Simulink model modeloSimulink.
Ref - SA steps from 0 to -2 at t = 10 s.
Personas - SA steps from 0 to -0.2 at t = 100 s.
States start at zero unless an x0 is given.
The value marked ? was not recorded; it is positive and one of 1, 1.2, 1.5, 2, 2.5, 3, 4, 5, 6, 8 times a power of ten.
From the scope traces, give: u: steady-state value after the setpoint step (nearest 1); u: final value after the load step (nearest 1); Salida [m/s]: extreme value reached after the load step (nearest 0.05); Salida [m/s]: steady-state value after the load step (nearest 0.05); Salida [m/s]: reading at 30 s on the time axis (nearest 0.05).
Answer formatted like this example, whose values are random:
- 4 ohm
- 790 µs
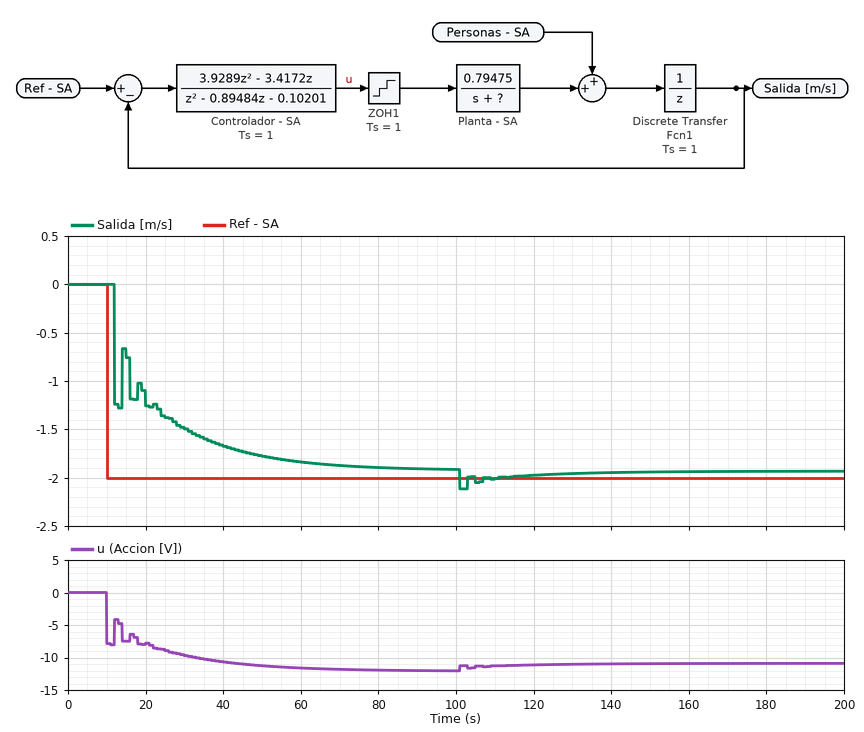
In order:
- -12
- -11
- -2.10
- -1.95
- -1.50
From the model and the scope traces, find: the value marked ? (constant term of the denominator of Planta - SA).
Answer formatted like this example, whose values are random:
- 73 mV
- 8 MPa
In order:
- 5
